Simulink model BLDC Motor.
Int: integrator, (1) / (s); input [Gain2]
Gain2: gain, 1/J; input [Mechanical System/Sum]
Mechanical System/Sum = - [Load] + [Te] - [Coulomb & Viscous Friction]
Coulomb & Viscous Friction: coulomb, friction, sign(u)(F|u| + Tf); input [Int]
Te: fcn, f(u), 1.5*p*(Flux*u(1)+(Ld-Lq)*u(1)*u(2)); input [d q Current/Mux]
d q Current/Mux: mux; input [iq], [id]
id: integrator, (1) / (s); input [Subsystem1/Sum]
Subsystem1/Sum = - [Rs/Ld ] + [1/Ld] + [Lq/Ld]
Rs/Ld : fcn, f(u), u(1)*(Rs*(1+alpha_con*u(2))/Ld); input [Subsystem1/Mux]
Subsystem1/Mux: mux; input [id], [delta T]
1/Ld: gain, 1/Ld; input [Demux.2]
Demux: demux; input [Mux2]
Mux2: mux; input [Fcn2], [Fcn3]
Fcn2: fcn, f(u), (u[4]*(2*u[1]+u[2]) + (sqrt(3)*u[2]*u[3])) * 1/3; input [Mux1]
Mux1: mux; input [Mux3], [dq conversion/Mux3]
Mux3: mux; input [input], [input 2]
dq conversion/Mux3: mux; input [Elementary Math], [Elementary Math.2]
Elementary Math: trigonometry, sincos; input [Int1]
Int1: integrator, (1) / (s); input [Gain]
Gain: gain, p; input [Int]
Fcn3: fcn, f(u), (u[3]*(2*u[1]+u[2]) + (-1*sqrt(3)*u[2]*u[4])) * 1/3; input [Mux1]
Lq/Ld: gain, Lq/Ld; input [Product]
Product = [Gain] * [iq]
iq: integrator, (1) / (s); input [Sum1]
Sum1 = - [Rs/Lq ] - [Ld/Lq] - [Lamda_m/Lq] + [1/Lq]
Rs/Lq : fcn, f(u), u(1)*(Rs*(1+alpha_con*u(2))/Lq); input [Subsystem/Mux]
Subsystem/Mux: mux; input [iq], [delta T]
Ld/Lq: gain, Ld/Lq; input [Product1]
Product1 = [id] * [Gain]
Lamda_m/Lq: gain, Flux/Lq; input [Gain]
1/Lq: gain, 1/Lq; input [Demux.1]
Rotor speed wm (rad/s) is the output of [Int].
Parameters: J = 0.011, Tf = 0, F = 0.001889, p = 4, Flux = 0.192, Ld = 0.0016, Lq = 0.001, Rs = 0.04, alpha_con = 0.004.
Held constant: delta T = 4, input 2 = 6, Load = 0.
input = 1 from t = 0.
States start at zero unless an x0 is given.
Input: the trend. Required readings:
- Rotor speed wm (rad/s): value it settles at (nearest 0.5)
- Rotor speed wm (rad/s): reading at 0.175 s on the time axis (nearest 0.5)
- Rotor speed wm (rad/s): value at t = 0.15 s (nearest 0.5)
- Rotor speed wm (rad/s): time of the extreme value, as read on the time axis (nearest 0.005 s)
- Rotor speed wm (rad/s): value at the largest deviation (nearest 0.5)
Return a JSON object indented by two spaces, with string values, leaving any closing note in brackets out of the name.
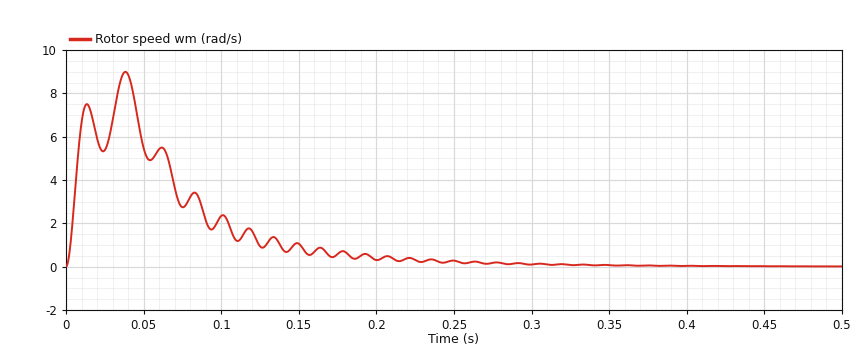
{
  "Rotor speed wm (rad/s): value it settles at": "0.0",
  "Rotor speed wm (rad/s): reading at 0.175 s on the time axis": "0.5",
  "Rotor speed wm (rad/s): value at t = 0.15 s": "1.0",
  "Rotor speed wm (rad/s): time of the extreme value, as read on the time axis": "0.040 s",
  "Rotor speed wm (rad/s): value at the largest deviation": "9.0"
}
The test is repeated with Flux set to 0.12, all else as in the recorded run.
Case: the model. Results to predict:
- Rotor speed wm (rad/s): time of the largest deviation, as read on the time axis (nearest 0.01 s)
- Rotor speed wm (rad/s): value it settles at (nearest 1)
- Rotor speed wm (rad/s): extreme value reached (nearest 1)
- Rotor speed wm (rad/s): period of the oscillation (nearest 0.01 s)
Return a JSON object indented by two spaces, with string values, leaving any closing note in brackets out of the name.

{
  "Rotor speed wm (rad/s): time of the largest deviation, as read on the time axis": "0.03 s",
  "Rotor speed wm (rad/s): value it settles at": "0",
  "Rotor speed wm (rad/s): extreme value reached": "17",
  "Rotor speed wm (rad/s): period of the oscillation": "0.04 s"
}
